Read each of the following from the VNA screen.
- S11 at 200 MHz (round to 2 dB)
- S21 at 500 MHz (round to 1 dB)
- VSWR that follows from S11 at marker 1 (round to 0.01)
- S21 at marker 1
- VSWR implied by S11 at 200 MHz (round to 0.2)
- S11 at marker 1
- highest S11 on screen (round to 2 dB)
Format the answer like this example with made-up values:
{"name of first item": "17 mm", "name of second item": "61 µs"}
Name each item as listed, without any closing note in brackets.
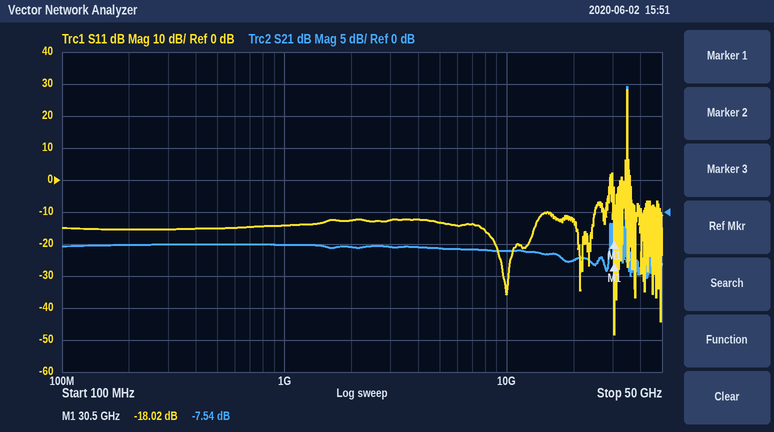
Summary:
{"S11 at 200 MHz": "-16 dB", "S21 at 500 MHz": "-5 dB", "VSWR that follows from S11 at marker 1": "1.29", "S21 at marker 1": "-7.54 dB", "VSWR implied by S11 at 200 MHz": "1.4", "S11 at marker 1": "-18.02 dB", "highest S11 on screen": "28 dB"}
